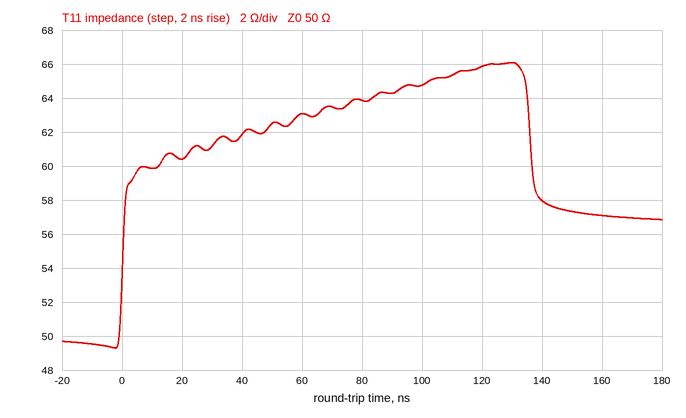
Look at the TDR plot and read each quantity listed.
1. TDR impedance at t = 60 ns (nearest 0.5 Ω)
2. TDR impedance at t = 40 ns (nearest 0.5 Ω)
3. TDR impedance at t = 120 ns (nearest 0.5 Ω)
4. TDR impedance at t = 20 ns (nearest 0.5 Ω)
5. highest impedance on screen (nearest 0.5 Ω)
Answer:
63.0 Ω
62.0 Ω
66.0 Ω
60.5 Ω
66.0 Ω
